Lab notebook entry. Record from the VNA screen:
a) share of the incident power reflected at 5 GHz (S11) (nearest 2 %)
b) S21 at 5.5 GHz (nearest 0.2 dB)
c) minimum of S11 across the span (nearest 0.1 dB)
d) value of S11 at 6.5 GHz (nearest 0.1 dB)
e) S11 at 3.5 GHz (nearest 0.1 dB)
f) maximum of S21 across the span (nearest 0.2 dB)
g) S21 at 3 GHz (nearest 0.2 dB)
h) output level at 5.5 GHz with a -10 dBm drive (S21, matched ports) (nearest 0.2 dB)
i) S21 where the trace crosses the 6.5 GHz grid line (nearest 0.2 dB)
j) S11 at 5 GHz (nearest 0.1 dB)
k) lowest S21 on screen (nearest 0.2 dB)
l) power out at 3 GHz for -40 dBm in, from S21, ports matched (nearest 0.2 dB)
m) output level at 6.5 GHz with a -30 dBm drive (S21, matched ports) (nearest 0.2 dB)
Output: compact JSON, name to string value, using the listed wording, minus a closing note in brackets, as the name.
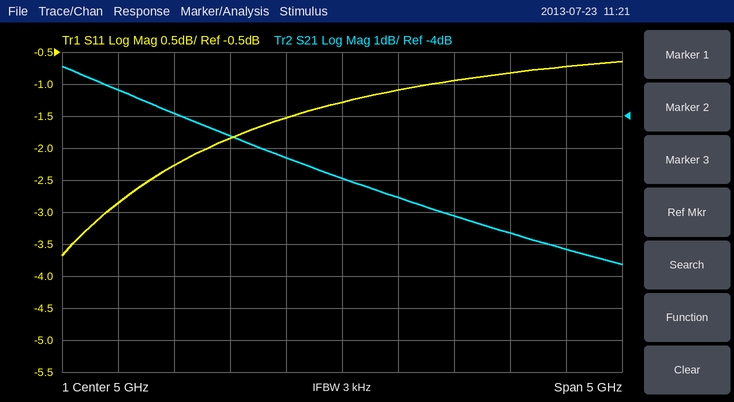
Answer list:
{"share of the incident power reflected at 5 GHz (S11)": "74 %", "S21 at 5.5 GHz": "-6.6 dB", "minimum of S11 across the span": "-3.7 dB", "value of S11 at 6.5 GHz": "-0.8 dB", "S11 at 3.5 GHz": "-2.3 dB", "maximum of S21 across the span": "-2.4 dB", "S21 at 3 GHz": "-3.2 dB", "output level at 5.5 GHz with a -10 dBm drive (S21, matched ports)": "-16.6 dBm", "S21 where the trace crosses the 6.5 GHz grid line": "-7.6 dB", "S11 at 5 GHz": "-1.3 dB", "lowest S21 on screen": "-8.6 dB", "power out at 3 GHz for -40 dBm in, from S21, ports matched": "-43.2 dBm", "output level at 6.5 GHz with a -30 dBm drive (S21, matched ports)": "-37.6 dBm"}
